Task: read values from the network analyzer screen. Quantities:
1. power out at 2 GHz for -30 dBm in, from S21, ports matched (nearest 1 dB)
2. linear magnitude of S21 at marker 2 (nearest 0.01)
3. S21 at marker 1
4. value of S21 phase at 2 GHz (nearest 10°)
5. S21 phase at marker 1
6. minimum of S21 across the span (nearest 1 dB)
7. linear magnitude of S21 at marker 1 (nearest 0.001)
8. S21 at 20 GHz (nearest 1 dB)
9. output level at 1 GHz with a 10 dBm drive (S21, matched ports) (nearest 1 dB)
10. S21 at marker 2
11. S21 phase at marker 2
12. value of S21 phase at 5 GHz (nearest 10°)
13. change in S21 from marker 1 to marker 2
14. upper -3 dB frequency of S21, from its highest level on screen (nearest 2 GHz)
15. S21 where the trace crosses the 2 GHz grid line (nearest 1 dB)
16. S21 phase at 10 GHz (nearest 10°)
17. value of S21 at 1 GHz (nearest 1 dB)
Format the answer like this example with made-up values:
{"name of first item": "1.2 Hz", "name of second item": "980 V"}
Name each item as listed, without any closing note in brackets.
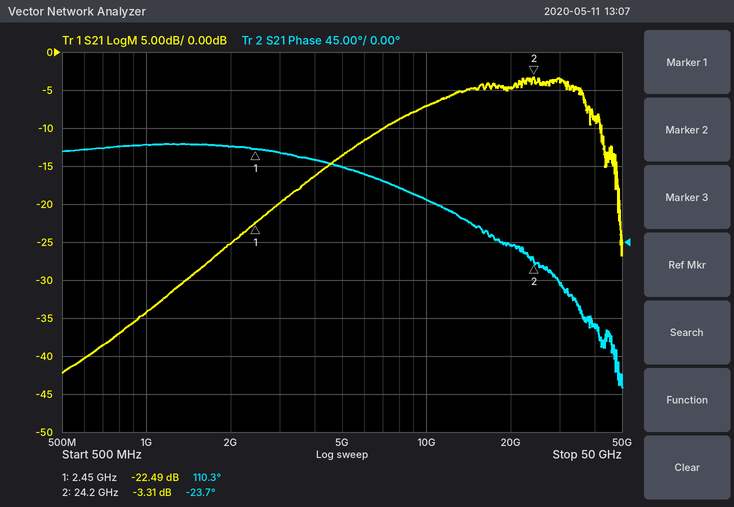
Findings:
{"power out at 2 GHz for -30 dBm in, from S21, ports matched": "-55 dBm", "linear magnitude of S21 at marker 2": "0.68", "S21 at marker 1": "-22.49 dB", "value of S21 phase at 2 GHz": "110°", "S21 phase at marker 1": "110.3°", "minimum of S21 across the span": "-42 dB", "linear magnitude of S21 at marker 1": "0.075", "S21 at 20 GHz": "-5 dB", "output level at 1 GHz with a 10 dBm drive (S21, matched ports)": "-24 dBm", "S21 at marker 2": "-3.31 dB", "S21 phase at marker 2": "-23.7°", "value of S21 phase at 5 GHz": "90°", "change in S21 from marker 1 to marker 2": "19.18 dB", "upper -3 dB frequency of S21, from its highest level on screen": "36 GHz", "S21 where the trace crosses the 2 GHz grid line": "-25 dB", "S21 phase at 10 GHz": "50°", "value of S21 at 1 GHz": "-34 dB"}
